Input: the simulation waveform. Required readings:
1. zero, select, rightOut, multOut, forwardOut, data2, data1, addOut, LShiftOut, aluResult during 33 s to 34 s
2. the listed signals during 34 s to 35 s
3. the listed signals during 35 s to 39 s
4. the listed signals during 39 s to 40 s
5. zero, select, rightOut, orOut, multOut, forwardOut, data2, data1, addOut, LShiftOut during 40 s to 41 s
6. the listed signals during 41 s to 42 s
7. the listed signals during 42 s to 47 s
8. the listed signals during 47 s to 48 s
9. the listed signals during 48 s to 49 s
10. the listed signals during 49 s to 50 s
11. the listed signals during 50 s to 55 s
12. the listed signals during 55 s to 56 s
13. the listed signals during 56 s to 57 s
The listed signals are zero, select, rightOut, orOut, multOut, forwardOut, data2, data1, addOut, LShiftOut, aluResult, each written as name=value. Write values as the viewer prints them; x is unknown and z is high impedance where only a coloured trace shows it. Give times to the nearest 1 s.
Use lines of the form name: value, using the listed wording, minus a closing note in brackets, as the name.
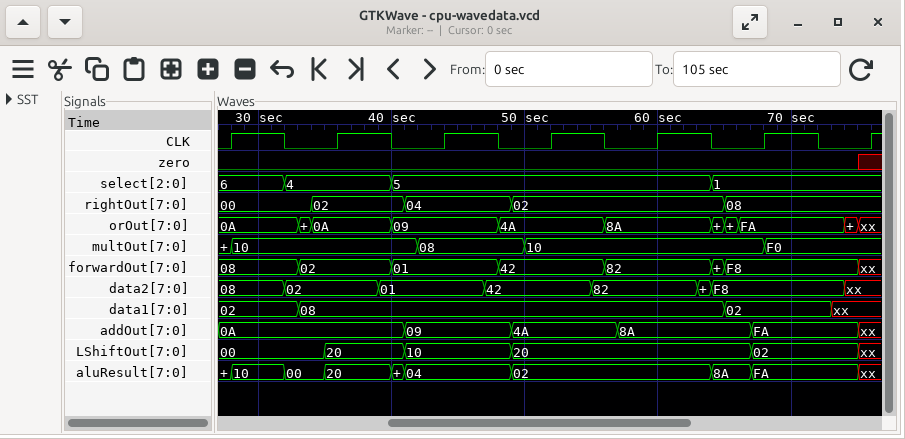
zero, select, rightOut, multOut, forwardOut, data2, data1, addOut, LShiftOut, aluResult during 33 s to 34 s: zero=0, select=4, rightOut=00, multOut=10, forwardOut=02, data2=02, data1=08, addOut=0A, LShiftOut=00, aluResult=00
the listed signals during 34 s to 35 s: zero=0, select=4, rightOut=02, orOut=0A, multOut=10, forwardOut=02, data2=02, data1=08, addOut=0A, LShiftOut=00, aluResult=00
the listed signals during 35 s to 39 s: zero=0, select=4, rightOut=02, orOut=0A, multOut=10, forwardOut=02, data2=02, data1=08, addOut=0A, LShiftOut=20, aluResult=20
the listed signals during 39 s to 40 s: zero=0, select=4, rightOut=02, orOut=0A, multOut=10, forwardOut=02, data2=01, data1=08, addOut=0A, LShiftOut=20, aluResult=20
zero, select, rightOut, orOut, multOut, forwardOut, data2, data1, addOut, LShiftOut during 40 s to 41 s: zero=0, select=5, rightOut=02, orOut=09, multOut=10, forwardOut=01, data2=01, data1=08, addOut=0A, LShiftOut=20
the listed signals during 41 s to 42 s: zero=0, select=5, rightOut=04, orOut=09, multOut=10, forwardOut=01, data2=01, data1=08, addOut=09, LShiftOut=10, aluResult=04
the listed signals during 42 s to 47 s: zero=0, select=5, rightOut=04, orOut=09, multOut=08, forwardOut=01, data2=01, data1=08, addOut=09, LShiftOut=10, aluResult=04
the listed signals during 47 s to 48 s: zero=0, select=5, rightOut=04, orOut=09, multOut=08, forwardOut=01, data2=42, data1=08, addOut=09, LShiftOut=10, aluResult=04
the listed signals during 48 s to 49 s: zero=0, select=5, rightOut=04, orOut=4A, multOut=08, forwardOut=42, data2=42, data1=08, addOut=09, LShiftOut=10, aluResult=04
the listed signals during 49 s to 50 s: zero=0, select=5, rightOut=02, orOut=4A, multOut=08, forwardOut=42, data2=42, data1=08, addOut=4A, LShiftOut=20, aluResult=02
the listed signals during 50 s to 55 s: zero=0, select=5, rightOut=02, orOut=4A, multOut=10, forwardOut=42, data2=42, data1=08, addOut=4A, LShiftOut=20, aluResult=02
the listed signals during 55 s to 56 s: zero=0, select=5, rightOut=02, orOut=4A, multOut=10, forwardOut=42, data2=82, data1=08, addOut=4A, LShiftOut=20, aluResult=02
the listed signals during 56 s to 57 s: zero=0, select=5, rightOut=02, orOut=8A, multOut=10, forwardOut=82, data2=82, data1=08, addOut=4A, LShiftOut=20, aluResult=02
